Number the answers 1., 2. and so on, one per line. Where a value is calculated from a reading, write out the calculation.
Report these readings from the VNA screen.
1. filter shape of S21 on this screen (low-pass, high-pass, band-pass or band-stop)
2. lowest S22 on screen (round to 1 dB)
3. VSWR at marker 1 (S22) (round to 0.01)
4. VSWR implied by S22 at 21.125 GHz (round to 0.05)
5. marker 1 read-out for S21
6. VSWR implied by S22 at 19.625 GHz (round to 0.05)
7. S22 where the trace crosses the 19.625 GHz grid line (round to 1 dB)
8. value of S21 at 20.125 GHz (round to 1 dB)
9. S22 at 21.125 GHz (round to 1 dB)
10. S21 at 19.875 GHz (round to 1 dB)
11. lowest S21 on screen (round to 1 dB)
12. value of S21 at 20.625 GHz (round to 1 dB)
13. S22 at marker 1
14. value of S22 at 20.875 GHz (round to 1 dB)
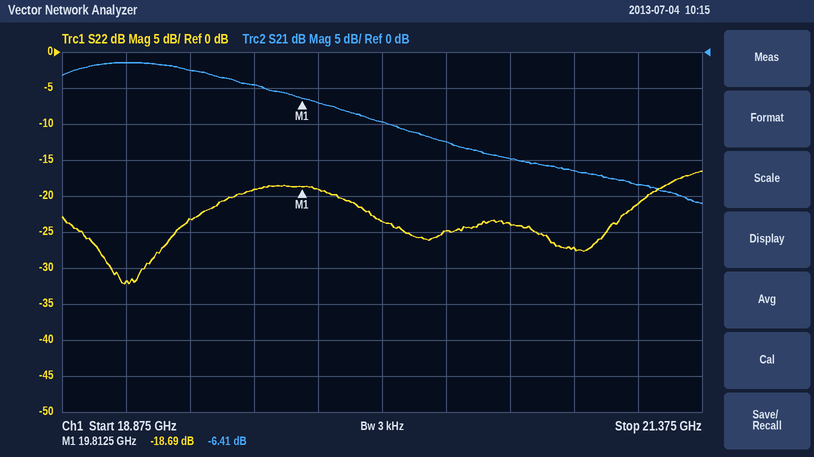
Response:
1. low-pass
2. -32 dB
3. (1 + 0.1163)/(1 − 0.1163) ≈ 1.26
4. |Γ| = 10^(-21/20) = 0.0891; VSWR = (1 + 0.0891)/(1 − 0.0891) ≈ 1.20
5. -6.41 dB
6. |Γ| = 10^(-19/20) = 0.1122; VSWR = (1 + 0.1122)/(1 − 0.1122) ≈ 1.25
7. -19 dB
8. -10 dB
9. -21 dB
10. -7 dB
11. -21 dB
12. -15 dB
13. -18.69 dB
14. -27 dB
